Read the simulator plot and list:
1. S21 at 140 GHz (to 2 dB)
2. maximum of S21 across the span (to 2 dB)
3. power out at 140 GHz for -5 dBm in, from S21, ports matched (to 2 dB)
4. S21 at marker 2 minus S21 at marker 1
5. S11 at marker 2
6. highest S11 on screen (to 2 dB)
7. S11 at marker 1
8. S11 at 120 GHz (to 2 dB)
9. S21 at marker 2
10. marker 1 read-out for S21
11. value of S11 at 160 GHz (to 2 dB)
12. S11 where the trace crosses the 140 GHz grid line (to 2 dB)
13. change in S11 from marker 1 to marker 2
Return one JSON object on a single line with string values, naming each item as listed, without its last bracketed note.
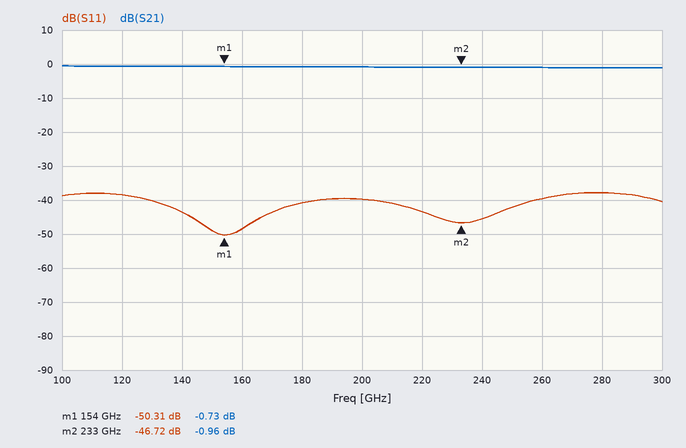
{"S21 at 140 GHz": "0 dB", "maximum of S21 across the span": "0 dB", "power out at 140 GHz for -5 dBm in, from S21, ports matched": "-6 dBm", "S21 at marker 2 minus S21 at marker 1": "-0.23 dB", "S11 at marker 2": "-46.72 dB", "highest S11 on screen": "-38 dB", "S11 at marker 1": "-50.31 dB", "S11 at 120 GHz": "-38 dB", "S21 at marker 2": "-0.96 dB", "marker 1 read-out for S21": "-0.73 dB", "value of S11 at 160 GHz": "-48 dB", "S11 where the trace crosses the 140 GHz grid line": "-44 dB", "change in S11 from marker 1 to marker 2": "3.59 dB"}
